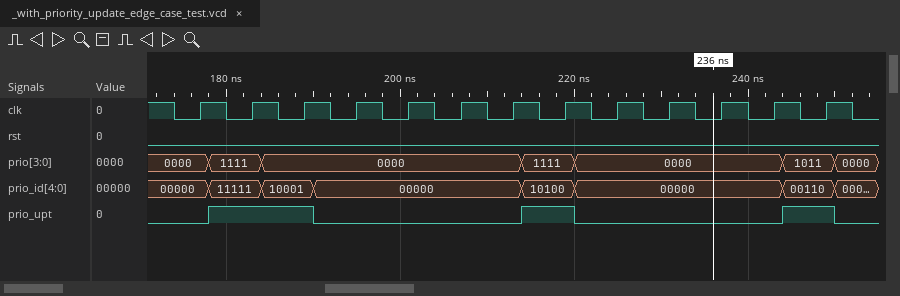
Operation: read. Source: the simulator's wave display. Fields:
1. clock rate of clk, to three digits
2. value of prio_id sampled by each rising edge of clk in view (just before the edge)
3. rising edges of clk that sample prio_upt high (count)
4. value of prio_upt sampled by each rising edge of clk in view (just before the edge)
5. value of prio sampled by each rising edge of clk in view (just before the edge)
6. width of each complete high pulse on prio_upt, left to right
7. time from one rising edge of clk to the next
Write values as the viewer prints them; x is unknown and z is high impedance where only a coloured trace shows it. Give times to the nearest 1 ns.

167 MHz
00000, 11111, 10001, 00000, 00000, 00000, 00000, 10100, 00000, 00000, 00000, 00000, 00110
4
0 1 1 0 0 0 0 1 0 0 0 0 1
0000, 1111, 0000, 0000, 0000, 0000, 0000, 1111, 0000, 0000, 0000, 0000, 1011
12 ns, 6 ns, 6 ns
6 ns
